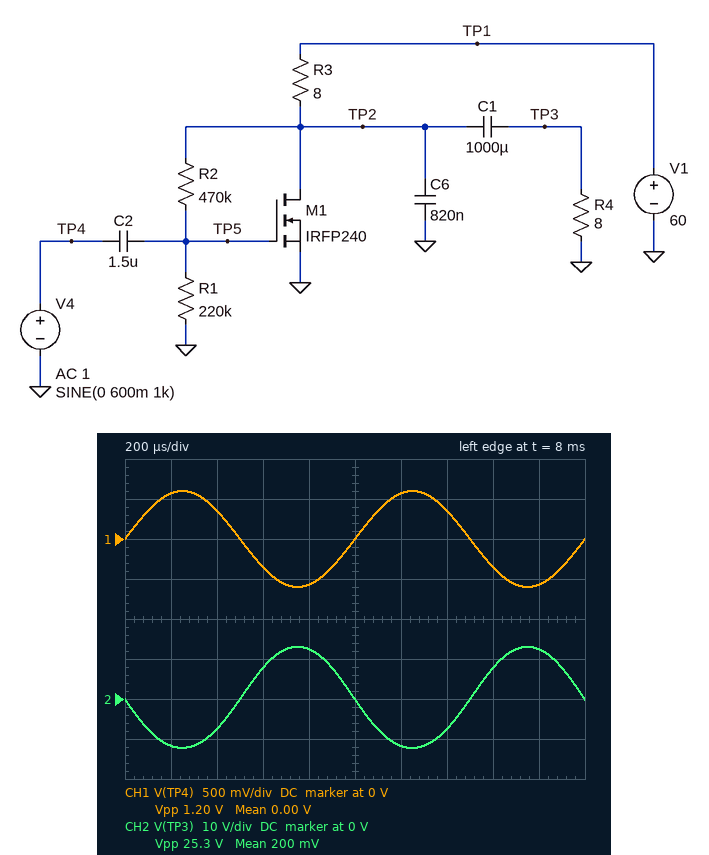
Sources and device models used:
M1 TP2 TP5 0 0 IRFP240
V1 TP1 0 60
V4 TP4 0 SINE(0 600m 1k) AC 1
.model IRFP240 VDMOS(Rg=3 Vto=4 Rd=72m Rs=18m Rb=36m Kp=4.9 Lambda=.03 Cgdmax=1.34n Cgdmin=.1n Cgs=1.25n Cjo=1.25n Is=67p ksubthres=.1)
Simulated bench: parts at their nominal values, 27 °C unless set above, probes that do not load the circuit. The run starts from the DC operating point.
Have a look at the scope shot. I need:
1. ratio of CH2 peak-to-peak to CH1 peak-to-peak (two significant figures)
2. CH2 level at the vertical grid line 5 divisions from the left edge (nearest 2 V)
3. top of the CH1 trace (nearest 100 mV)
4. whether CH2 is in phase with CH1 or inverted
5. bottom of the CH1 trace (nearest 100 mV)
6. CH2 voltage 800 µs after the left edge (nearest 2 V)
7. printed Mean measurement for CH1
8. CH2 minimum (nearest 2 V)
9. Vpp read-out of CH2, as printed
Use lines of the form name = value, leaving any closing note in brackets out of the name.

ratio of CH2 peak-to-peak to CH1 peak-to-peak = 21
CH2 level at the vertical grid line 5 divisions from the left edge = 0 V
top of the CH1 trace = 600 mV
whether CH2 is in phase with CH1 or inverted = inverted
bottom of the CH1 trace = -600 mV
CH2 voltage 800 µs after the left edge = 12 V
printed Mean measurement for CH1 = 0.00 V
CH2 minimum = -12 V
Vpp read-out of CH2, as printed = 25.3 V
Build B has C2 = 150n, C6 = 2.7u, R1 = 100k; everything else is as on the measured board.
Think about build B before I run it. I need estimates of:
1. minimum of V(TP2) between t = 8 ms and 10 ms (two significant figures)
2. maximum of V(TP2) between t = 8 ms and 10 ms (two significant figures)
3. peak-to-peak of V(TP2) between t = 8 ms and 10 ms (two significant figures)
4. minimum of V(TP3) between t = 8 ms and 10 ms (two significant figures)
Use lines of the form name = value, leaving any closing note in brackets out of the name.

minimum of V(TP2) between t = 8 ms and 10 ms = 15 V
maximum of V(TP2) between t = 8 ms and 10 ms = 41 V
peak-to-peak of V(TP2) between t = 8 ms and 10 ms = 26 V
minimum of V(TP3) between t = 8 ms and 10 ms = -13 V
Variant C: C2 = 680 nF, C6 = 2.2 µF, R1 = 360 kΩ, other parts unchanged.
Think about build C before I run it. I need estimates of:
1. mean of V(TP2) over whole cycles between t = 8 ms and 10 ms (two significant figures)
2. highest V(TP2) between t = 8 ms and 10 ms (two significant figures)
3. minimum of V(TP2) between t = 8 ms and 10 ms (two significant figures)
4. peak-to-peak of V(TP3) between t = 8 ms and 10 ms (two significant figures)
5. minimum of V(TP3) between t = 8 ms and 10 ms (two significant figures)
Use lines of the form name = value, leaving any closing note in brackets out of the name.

mean of V(TP2) over whole cycles between t = 8 ms and 10 ms = 13 V
highest V(TP2) between t = 8 ms and 10 ms = 25 V
minimum of V(TP2) between t = 8 ms and 10 ms = 2.2 V
peak-to-peak of V(TP3) between t = 8 ms and 10 ms = 23 V
minimum of V(TP3) between t = 8 ms and 10 ms = -11 V
